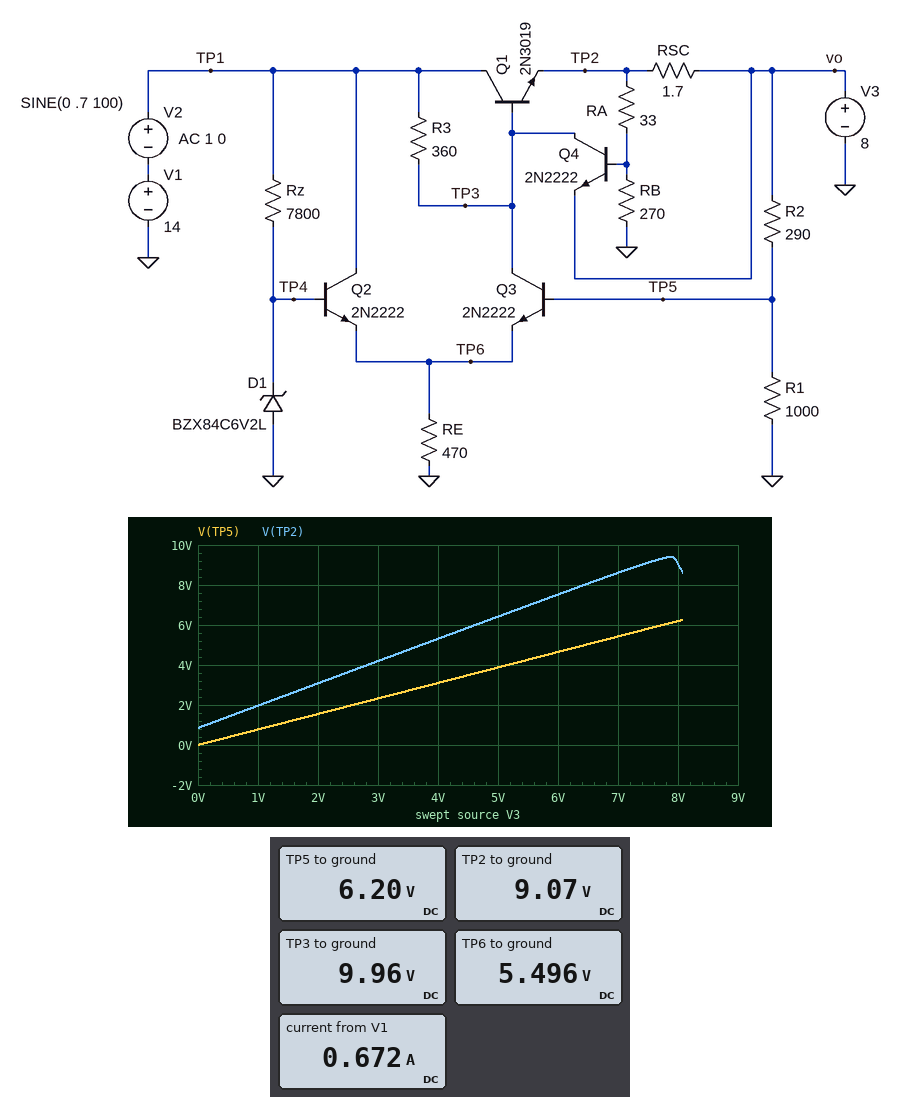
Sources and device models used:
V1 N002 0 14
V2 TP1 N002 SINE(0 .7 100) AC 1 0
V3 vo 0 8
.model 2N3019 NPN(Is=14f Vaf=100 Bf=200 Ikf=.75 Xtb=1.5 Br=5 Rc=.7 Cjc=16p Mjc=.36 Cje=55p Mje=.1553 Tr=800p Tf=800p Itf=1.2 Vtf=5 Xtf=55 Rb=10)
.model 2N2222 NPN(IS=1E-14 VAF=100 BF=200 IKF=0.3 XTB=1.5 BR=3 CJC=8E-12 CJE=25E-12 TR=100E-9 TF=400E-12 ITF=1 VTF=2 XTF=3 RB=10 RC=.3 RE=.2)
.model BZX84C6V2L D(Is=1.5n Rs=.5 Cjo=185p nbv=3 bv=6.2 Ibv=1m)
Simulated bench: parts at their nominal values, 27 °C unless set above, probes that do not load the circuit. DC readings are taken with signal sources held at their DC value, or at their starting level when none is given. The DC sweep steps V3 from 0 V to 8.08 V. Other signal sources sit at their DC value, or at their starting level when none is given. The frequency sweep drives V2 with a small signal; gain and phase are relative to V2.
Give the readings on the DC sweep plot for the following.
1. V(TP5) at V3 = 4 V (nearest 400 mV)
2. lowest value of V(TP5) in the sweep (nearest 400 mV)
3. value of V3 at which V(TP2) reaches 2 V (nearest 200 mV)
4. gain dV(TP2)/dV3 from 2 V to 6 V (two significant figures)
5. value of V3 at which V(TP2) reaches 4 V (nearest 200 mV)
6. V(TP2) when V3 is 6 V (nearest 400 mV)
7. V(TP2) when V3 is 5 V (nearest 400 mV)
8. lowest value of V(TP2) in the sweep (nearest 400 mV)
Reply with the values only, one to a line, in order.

3.2 V
0 V
1.0 V
1.1 V/V
2.8 V
7.6 V
6.4 V
800 mV
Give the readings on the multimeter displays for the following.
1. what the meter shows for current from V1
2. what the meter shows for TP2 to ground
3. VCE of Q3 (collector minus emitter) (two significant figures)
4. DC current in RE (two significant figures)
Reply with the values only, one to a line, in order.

0.672 A
9.07 V
4.5 V
12 mA
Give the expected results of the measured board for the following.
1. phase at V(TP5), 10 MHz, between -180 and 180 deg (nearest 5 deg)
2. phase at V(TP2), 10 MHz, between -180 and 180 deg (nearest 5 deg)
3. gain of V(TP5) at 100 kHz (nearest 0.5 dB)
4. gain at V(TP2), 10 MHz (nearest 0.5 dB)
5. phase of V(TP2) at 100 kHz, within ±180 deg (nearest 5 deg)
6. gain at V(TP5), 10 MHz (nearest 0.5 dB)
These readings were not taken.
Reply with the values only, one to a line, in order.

75 deg
-5 deg
-58.5 dB
-23.5 dB
-25 deg
-37.0 dB
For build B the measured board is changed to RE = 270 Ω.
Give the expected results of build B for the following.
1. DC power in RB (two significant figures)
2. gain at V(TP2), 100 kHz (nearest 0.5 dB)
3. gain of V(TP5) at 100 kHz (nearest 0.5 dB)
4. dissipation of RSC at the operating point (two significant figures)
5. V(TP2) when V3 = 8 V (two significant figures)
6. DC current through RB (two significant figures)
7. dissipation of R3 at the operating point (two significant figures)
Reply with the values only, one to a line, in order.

220 mW
-7.5 dB
-55.0 dB
290 mW
8.7 V
29 mA
55 mW
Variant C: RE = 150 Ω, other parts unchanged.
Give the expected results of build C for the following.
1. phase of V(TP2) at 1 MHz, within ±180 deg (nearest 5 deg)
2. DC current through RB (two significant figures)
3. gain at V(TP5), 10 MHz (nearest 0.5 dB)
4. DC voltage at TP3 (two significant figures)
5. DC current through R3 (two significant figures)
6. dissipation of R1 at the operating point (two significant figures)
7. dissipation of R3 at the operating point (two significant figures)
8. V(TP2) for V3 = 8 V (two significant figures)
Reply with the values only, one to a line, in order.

20 deg
26 mA
-32.5 dB
8.5 V
15 mA
38 mW
85 mW
8.0 V
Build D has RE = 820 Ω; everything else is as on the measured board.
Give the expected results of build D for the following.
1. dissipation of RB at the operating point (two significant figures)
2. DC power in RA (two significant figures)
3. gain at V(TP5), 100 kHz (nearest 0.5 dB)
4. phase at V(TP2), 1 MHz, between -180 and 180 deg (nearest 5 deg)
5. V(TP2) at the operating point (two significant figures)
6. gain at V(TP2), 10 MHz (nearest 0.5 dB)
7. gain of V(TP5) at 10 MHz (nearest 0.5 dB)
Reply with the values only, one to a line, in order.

250 mW
31 mW
-62.5 dB
-20 deg
9.3 V
-22.0 dB
-37.5 dB
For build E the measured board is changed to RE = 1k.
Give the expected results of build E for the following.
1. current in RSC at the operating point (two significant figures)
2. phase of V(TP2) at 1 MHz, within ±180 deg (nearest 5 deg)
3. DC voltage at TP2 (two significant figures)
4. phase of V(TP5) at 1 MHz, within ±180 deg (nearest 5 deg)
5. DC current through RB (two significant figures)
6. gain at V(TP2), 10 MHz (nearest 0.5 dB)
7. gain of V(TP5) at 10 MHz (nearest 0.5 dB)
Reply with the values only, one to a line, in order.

770 mA
-15 deg
9.3 V
60 deg
31 mA
-22.0 dB
-37.5 dB
